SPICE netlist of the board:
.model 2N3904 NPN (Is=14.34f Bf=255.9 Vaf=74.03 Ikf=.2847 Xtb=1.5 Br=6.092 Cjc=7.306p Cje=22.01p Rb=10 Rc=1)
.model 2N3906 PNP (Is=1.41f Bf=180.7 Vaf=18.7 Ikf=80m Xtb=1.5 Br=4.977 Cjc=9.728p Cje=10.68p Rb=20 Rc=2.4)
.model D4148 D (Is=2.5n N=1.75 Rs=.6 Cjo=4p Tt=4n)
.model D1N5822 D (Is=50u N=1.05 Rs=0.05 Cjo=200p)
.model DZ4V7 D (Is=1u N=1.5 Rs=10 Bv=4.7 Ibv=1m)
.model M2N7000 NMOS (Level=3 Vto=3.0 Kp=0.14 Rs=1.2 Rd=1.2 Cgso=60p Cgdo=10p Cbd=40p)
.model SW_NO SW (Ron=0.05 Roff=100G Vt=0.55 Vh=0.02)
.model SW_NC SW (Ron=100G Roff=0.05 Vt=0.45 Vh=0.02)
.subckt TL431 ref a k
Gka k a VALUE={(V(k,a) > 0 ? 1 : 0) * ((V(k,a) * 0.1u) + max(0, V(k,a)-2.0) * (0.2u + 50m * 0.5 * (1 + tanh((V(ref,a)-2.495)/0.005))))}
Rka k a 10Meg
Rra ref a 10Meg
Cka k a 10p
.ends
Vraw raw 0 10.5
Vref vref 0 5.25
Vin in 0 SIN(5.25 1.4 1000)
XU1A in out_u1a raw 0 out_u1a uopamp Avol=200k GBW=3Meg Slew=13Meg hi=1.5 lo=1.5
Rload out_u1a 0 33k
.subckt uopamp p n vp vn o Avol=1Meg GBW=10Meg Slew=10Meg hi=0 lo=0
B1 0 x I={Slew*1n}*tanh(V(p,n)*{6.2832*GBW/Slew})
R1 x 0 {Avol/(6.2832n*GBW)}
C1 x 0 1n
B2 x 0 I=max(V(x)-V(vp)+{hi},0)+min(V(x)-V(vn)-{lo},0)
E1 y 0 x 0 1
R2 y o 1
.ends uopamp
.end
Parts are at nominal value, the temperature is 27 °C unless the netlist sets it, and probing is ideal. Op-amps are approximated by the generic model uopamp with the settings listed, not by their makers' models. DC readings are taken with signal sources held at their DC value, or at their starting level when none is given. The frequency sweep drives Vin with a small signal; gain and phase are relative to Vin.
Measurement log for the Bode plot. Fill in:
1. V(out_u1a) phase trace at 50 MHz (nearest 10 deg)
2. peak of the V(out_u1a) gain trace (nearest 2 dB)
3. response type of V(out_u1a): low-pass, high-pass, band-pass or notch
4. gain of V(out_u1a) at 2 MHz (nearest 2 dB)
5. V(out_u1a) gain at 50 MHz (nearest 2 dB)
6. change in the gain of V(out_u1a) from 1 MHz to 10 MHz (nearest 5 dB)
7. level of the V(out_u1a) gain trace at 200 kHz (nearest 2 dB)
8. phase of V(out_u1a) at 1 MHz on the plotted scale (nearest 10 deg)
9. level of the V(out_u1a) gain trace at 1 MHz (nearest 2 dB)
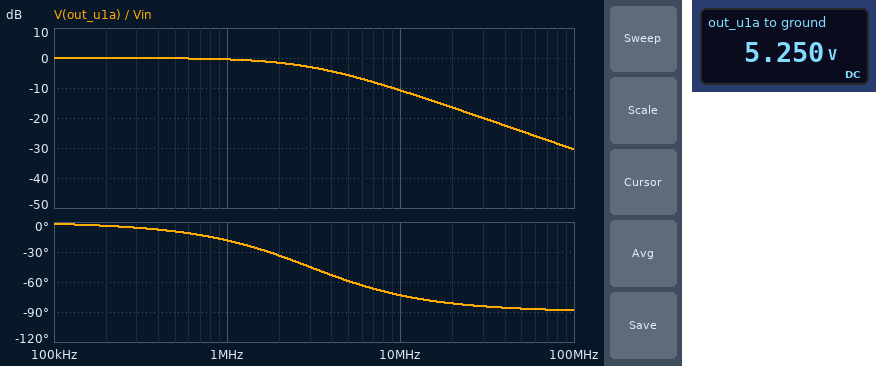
-90 deg
0 dB
low-pass
-2 dB
-24 dB
-10 dB
0 dB
-20 deg
0 dB
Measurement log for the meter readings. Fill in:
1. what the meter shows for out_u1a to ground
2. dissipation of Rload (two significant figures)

5.250 V
840 µW
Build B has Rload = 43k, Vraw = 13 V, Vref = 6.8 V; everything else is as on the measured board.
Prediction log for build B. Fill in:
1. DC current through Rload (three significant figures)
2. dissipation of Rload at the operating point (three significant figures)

122 µA
641 µW
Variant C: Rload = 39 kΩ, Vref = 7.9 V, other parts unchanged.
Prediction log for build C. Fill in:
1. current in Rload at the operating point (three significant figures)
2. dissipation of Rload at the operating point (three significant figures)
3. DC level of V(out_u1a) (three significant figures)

135 µA
707 µW
5.25 V
